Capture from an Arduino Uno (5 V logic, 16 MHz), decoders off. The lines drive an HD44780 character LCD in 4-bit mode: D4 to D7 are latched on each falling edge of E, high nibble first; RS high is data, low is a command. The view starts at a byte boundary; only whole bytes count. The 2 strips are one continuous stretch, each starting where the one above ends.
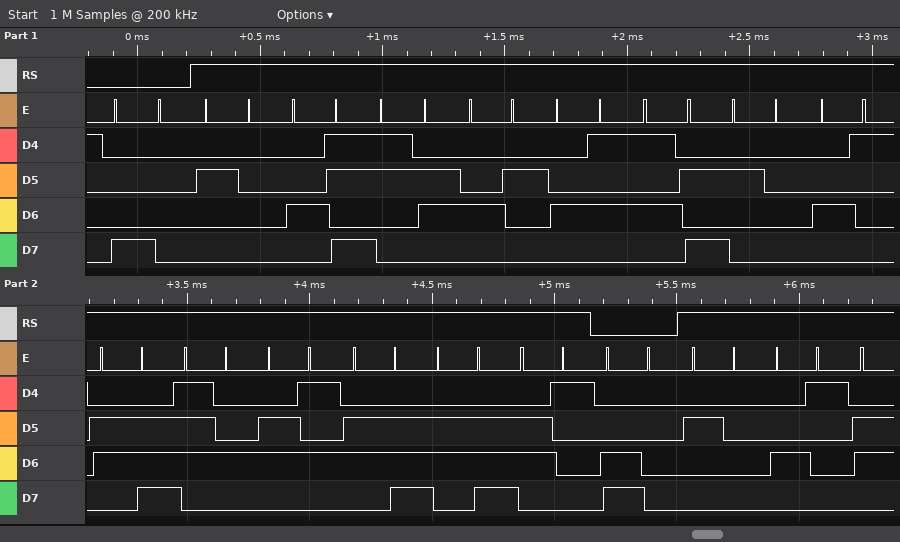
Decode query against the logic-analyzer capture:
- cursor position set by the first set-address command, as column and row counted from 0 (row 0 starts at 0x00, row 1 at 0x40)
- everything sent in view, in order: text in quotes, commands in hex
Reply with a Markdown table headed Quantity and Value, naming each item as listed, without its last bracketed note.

| Quantity | Value |
|---|---|
| cursor position set by the first set-address command, as column and row counted from 0 | column 0, row 0 |
| everything sent in view, in order: text in quotes, commands in hex | 0x80 " K6BEZ Antenna" 0xC0 " A" |
